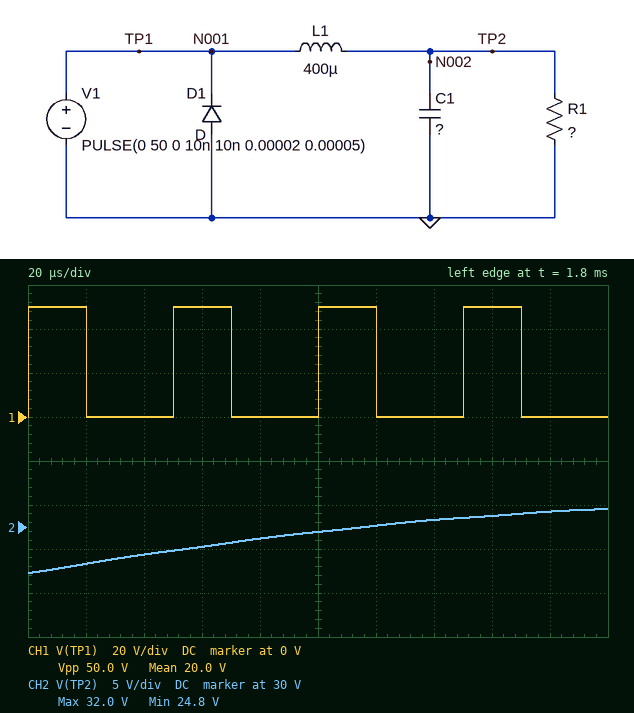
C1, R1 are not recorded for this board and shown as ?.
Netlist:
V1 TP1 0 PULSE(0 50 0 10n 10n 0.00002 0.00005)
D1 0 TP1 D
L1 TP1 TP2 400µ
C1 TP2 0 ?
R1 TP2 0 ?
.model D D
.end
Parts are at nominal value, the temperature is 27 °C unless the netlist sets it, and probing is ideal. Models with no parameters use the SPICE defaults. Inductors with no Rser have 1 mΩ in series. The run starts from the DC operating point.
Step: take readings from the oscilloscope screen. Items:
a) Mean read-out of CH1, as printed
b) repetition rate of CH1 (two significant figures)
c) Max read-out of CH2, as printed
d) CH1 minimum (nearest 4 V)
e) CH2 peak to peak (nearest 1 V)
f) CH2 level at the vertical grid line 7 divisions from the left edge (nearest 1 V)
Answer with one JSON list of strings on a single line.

["20.0 V", "20 kHz", "32.0 V", "0 V", "7 V", "31 V"]
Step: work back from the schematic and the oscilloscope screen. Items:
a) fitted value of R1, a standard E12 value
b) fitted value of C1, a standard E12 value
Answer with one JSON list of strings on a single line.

["18 Ω", "120 µF"]
